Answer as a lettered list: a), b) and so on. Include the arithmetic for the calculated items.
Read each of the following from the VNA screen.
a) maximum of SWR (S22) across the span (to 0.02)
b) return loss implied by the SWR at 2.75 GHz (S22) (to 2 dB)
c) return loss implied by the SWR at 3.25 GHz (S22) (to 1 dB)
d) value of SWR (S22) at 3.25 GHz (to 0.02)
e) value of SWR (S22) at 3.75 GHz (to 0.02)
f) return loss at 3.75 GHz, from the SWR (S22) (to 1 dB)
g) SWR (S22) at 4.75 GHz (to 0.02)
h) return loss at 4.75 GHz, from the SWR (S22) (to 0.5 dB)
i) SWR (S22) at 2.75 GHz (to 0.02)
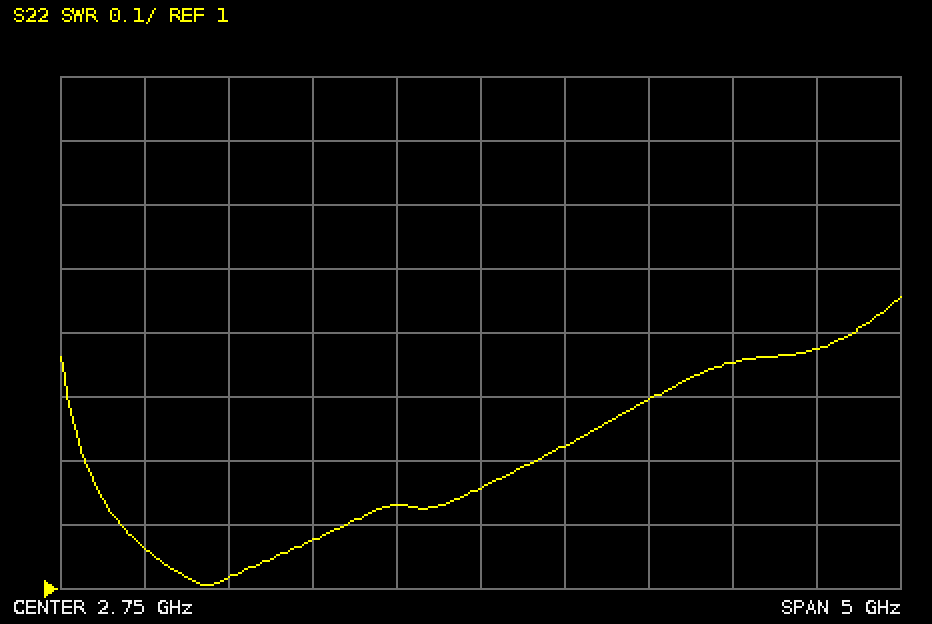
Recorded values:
a) 1.46
b) −20 log10((1.16 − 1)/(1.16 + 1)) ≈ 22.6 dB, so 22 dB to the nearest 2 dB
c) −20 log10((1.22 − 1)/(1.22 + 1)) ≈ 20 dB
d) 1.22
e) 1.30
f) −20 log10((1.3 − 1)/(1.3 + 1)) ≈ 18 dB
g) 1.38
h) −20 log10((1.38 − 1)/(1.38 + 1)) ≈ 15.9 dB, so 16.0 dB to the nearest 0.5 dB
i) 1.16
